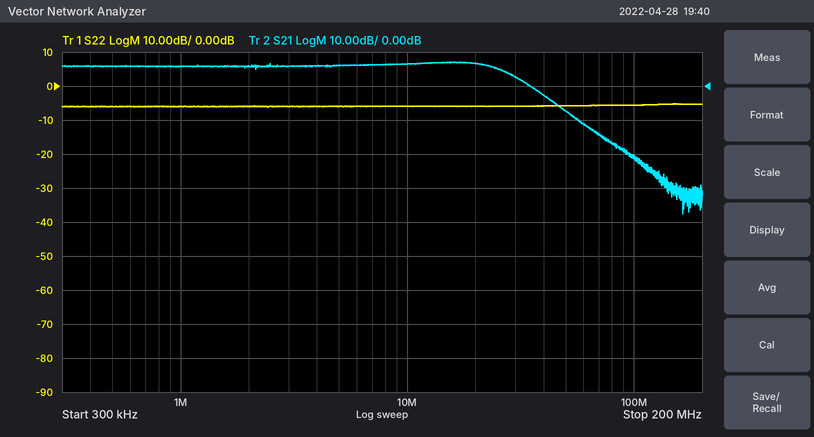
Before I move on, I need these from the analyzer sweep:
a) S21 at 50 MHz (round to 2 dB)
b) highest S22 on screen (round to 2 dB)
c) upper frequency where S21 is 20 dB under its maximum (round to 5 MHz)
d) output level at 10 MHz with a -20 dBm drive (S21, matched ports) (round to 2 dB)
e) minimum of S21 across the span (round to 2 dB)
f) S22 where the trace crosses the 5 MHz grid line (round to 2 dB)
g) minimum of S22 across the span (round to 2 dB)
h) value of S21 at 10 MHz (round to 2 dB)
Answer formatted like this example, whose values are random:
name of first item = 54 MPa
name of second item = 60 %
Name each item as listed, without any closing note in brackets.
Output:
S21 at 50 MHz = -8 dB
highest S22 on screen = -6 dB
upper frequency where S21 is 20 dB under its maximum = 65 MHz
output level at 10 MHz with a -20 dBm drive (S21, matched ports) = -14 dBm
minimum of S21 across the span = -38 dB
S22 where the trace crosses the 5 MHz grid line = -6 dB
minimum of S22 across the span = -6 dB
value of S21 at 10 MHz = 6 dB
